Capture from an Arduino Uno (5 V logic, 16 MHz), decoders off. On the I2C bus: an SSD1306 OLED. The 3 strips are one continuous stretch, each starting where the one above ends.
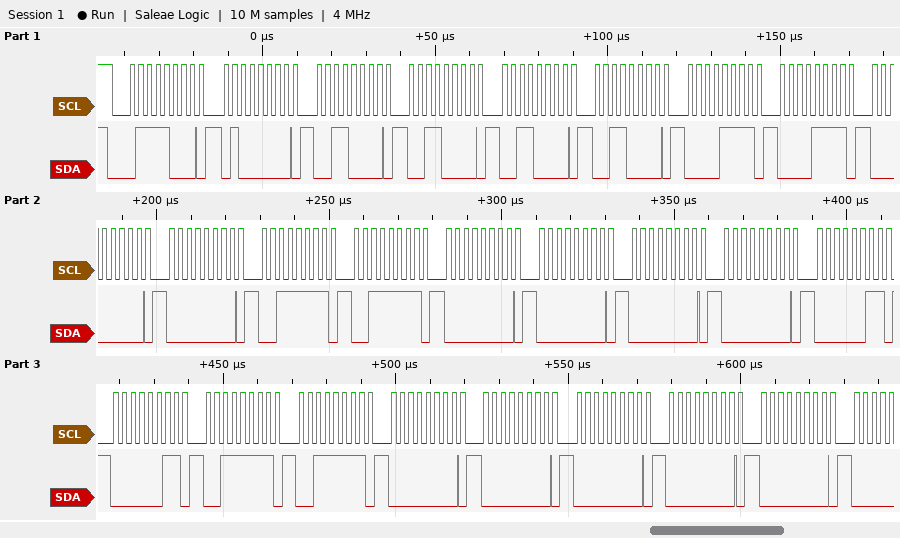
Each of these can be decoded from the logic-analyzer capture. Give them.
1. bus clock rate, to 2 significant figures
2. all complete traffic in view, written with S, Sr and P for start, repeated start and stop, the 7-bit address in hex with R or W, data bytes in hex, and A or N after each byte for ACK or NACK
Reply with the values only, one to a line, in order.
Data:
400 kHz
S 3CW A 40 A 30 A 30 A 30 A 30 A 0F A 0F A 00 A 00 A 3F A 3F A 00 A 00 A 00 A 00 A 03 A 03 A 3F A 3F A 00 A 00 A 00 A 00 A 00 A
